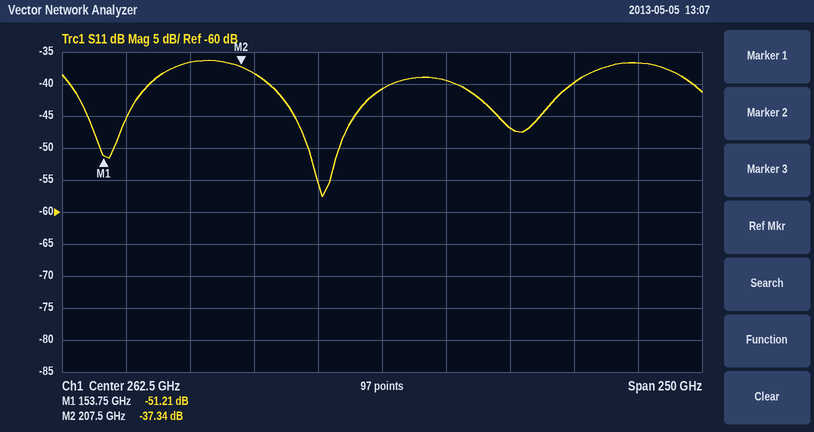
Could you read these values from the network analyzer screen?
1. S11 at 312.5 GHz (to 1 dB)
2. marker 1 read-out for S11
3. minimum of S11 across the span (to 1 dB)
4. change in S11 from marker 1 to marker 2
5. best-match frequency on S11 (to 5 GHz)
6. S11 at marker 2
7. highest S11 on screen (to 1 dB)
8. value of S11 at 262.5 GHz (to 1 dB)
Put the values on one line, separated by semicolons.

-47 dB; -51.21 dB; -58 dB; 13.87 dB; 240 GHz; -37.34 dB; -36 dB; -41 dB
